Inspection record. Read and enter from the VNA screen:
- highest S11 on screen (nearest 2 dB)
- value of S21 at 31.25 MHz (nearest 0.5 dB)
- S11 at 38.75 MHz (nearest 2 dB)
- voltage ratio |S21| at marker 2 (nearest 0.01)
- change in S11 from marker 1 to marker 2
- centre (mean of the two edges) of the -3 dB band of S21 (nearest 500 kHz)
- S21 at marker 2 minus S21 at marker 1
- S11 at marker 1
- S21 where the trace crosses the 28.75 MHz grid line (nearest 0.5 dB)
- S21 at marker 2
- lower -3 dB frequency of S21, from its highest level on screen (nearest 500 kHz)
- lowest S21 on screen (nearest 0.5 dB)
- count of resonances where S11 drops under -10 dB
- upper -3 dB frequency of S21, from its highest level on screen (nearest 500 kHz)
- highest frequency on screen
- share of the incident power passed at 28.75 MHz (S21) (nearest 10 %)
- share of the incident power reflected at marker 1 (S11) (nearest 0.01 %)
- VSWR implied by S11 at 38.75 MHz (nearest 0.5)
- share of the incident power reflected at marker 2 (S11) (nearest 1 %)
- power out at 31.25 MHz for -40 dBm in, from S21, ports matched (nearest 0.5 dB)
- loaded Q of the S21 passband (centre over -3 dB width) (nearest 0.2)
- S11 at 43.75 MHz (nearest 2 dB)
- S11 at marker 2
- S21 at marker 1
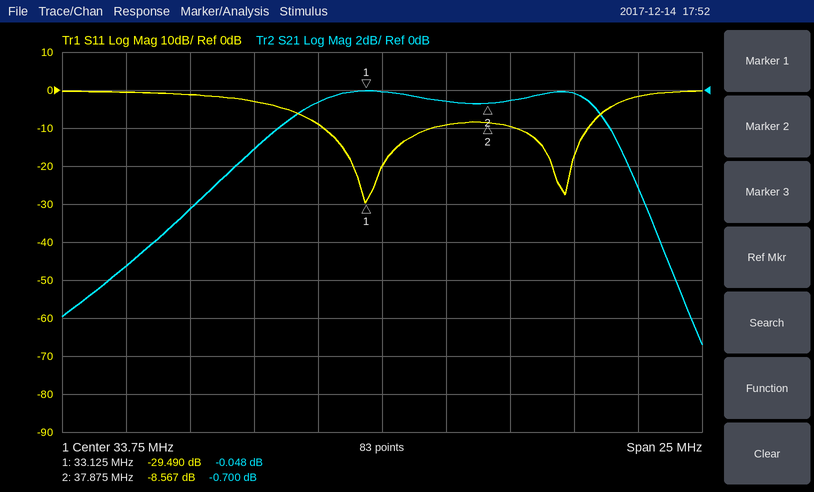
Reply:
0 dB
-0.5 dB
-10 dB
0.92
20.923 dB
36.0 MHz
-0.652 dB
-29.490 dB
-3.0 dB
-0.700 dB
29.0 MHz
-13.5 dB
2
43.0 MHz
46.25 MHz
50 %
0.11 %
2.0
14 %
-40.5 dBm
2.6
-2 dB
-8.567 dB
-0.048 dB
